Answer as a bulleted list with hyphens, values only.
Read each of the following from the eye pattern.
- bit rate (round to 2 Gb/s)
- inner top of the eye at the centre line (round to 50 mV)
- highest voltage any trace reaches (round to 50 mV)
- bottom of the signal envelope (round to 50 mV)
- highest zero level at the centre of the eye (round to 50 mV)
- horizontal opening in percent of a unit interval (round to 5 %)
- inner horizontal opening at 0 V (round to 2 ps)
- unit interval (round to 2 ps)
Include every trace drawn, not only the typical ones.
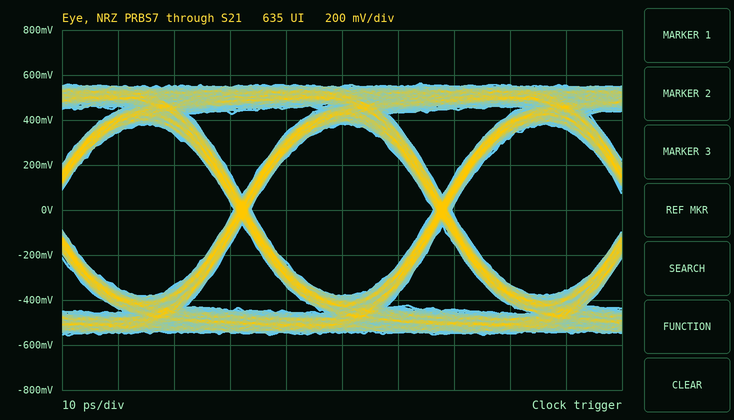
- 28 Gb/s
- 400 mV
- 550 mV
- -550 mV
- -400 mV
- 90 %
- 32 ps
- 36 ps
